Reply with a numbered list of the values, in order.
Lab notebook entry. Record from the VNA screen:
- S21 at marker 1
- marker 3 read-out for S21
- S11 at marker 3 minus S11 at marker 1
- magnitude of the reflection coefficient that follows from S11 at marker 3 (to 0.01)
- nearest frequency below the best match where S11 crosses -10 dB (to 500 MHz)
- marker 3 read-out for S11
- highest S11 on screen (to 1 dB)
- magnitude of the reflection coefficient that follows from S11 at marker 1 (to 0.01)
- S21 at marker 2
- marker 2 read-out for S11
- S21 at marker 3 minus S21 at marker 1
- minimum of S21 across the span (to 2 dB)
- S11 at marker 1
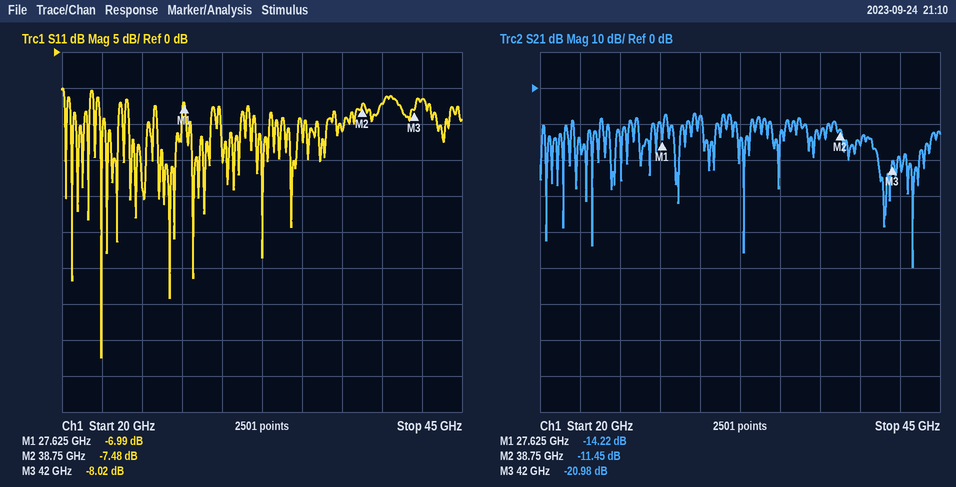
1. -14.22 dB
2. -20.98 dB
3. -1.03 dB
4. 0.40
5. 22.5 GHz
6. -8.02 dB
7. -5 dB
8. 0.45
9. -11.45 dB
10. -7.48 dB
11. -6.76 dB
12. -50 dB
13. -6.99 dB
